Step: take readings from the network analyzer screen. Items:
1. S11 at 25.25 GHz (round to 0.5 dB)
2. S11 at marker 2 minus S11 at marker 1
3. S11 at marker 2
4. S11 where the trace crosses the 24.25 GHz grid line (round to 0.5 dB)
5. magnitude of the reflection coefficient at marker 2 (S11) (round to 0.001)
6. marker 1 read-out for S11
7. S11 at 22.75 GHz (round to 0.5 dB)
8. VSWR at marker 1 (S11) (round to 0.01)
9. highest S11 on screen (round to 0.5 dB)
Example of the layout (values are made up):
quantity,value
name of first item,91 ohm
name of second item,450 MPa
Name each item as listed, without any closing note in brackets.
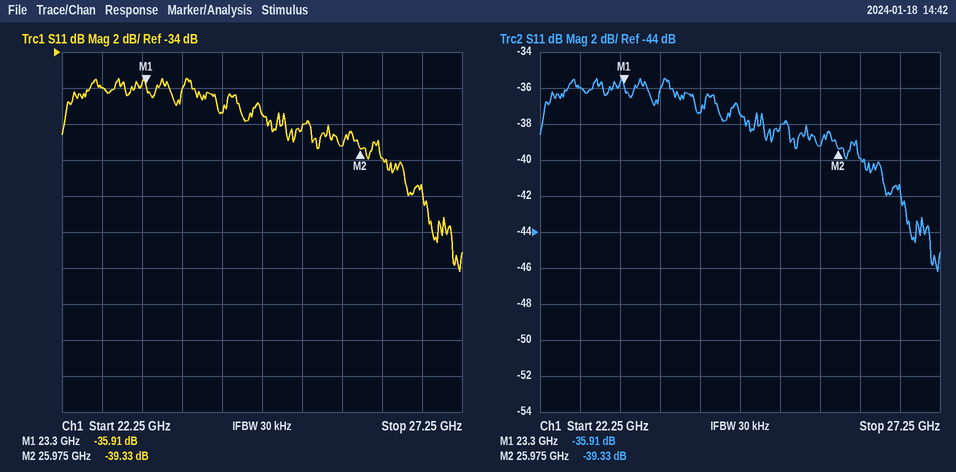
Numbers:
quantity,value
S11 at 25.25 GHz,-38.0 dB
S11 at marker 2 minus S11 at marker 1,-3.42 dB
S11 at marker 2,-39.33 dB
S11 where the trace crosses the 24.25 GHz grid line,-37.5 dB
magnitude of the reflection coefficient at marker 2 (S11),0.011
marker 1 read-out for S11,-35.91 dB
S11 at 22.75 GHz,-36.0 dB
VSWR at marker 1 (S11),1.03
highest S11 on screen,-35.5 dB
